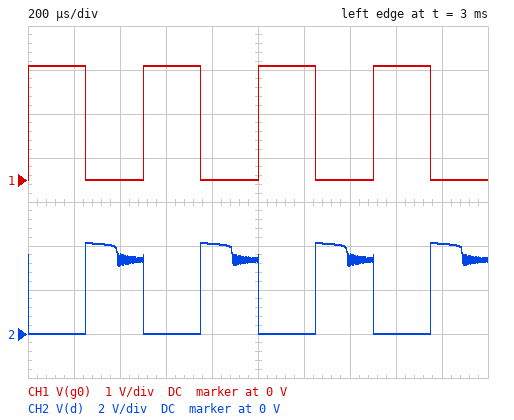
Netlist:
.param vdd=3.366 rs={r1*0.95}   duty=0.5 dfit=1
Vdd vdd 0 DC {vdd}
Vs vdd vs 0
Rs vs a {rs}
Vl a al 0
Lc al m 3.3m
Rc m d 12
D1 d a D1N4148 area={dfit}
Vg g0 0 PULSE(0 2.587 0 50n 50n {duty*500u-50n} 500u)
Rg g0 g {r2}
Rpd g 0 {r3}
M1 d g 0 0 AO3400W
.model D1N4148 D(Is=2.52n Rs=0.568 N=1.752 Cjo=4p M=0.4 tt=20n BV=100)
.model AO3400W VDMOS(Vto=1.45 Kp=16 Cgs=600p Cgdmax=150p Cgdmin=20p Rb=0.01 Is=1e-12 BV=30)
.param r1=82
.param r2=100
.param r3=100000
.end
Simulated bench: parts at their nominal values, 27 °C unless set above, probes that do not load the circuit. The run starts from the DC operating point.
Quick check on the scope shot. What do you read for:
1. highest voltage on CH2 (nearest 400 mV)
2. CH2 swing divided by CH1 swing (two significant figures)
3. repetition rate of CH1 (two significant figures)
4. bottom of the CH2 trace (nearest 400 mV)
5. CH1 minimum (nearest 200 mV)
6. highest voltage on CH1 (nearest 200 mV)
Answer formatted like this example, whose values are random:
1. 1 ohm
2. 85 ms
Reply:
1. 4.0 V
2. 1.6
3. 2.0 kHz
4. 0 V
5. 0 V
6. 2.6 V
